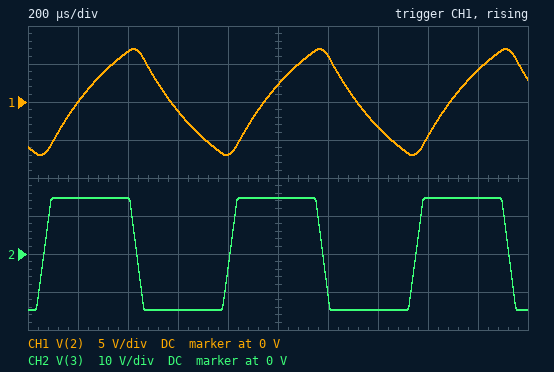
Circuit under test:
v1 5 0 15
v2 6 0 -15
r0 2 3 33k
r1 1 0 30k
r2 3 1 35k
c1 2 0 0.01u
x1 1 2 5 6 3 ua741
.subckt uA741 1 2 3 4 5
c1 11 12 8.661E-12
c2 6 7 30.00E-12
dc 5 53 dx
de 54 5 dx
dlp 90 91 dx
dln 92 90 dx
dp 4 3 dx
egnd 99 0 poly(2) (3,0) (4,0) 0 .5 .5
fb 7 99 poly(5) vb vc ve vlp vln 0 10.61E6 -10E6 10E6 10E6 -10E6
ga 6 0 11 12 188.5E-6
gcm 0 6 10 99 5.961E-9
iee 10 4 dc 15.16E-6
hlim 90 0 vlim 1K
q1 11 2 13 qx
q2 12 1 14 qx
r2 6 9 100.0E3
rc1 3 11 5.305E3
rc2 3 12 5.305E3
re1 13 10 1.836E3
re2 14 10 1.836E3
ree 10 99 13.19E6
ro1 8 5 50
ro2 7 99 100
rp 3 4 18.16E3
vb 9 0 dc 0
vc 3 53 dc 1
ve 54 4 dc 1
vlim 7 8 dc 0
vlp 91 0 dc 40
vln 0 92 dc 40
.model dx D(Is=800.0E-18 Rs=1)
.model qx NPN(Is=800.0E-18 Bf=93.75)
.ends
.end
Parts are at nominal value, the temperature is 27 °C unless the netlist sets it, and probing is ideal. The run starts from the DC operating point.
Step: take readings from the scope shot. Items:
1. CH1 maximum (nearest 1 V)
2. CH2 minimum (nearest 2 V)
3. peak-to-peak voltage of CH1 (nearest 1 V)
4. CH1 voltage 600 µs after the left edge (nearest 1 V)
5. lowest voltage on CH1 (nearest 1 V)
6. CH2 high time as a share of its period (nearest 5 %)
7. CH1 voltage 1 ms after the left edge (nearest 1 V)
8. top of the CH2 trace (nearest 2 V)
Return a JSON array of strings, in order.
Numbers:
["7 V", "-14 V", "14 V", "-1 V", "-7 V", "50 %", "2 V", "14 V"]
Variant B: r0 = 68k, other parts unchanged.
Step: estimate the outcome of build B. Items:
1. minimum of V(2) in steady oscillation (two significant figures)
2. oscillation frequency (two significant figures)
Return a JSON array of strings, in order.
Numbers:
["-6.9 V", "690 Hz"]
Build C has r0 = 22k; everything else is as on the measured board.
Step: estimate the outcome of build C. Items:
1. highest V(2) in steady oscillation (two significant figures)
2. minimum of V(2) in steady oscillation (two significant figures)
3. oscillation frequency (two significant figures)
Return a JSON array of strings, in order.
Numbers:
["7.1 V", "-7.1 V", "1.9 kHz"]
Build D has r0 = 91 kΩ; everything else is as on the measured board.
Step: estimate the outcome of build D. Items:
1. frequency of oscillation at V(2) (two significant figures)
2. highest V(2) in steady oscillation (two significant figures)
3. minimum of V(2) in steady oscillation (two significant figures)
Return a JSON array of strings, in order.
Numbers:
["530 Hz", "6.8 V", "-6.8 V"]
